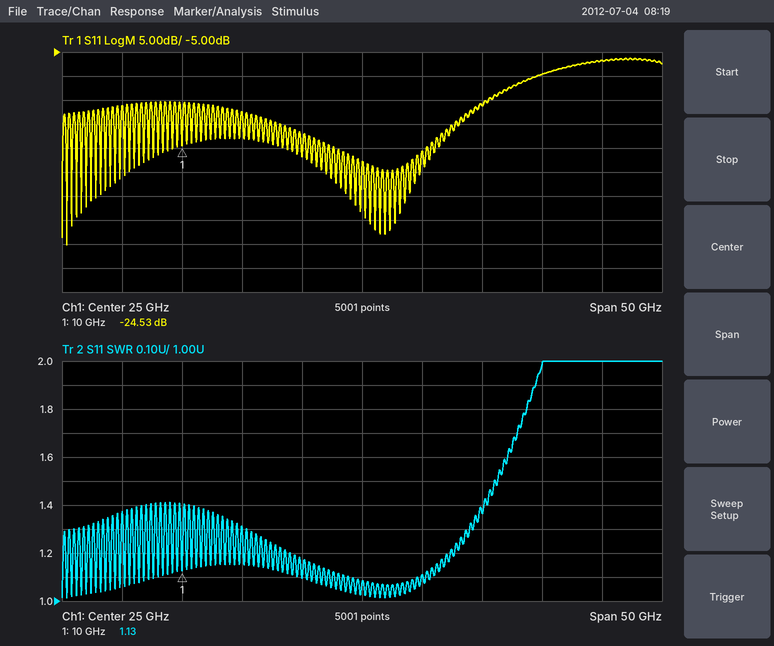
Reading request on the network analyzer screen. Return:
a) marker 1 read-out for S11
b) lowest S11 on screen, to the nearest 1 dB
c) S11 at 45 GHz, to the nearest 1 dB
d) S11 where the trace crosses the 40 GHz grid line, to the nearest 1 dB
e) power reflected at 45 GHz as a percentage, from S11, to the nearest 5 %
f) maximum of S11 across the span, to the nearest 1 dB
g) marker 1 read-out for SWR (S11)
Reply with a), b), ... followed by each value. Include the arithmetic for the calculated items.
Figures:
a) -24.53 dB
b) -45 dB
c) -7 dB
d) -10 dB
e) 10^(-7/10) ≈ 20 %
f) -6 dB
g) 1.13
